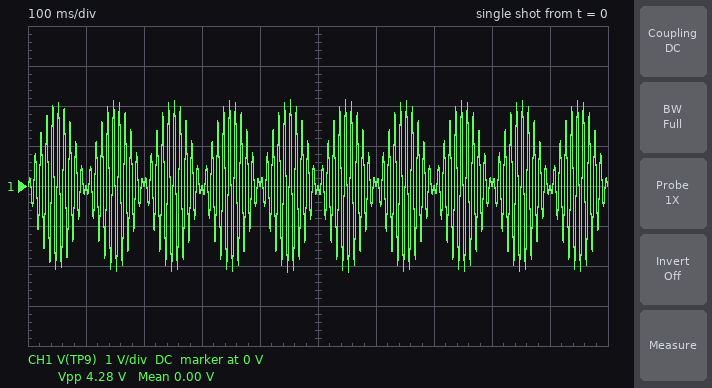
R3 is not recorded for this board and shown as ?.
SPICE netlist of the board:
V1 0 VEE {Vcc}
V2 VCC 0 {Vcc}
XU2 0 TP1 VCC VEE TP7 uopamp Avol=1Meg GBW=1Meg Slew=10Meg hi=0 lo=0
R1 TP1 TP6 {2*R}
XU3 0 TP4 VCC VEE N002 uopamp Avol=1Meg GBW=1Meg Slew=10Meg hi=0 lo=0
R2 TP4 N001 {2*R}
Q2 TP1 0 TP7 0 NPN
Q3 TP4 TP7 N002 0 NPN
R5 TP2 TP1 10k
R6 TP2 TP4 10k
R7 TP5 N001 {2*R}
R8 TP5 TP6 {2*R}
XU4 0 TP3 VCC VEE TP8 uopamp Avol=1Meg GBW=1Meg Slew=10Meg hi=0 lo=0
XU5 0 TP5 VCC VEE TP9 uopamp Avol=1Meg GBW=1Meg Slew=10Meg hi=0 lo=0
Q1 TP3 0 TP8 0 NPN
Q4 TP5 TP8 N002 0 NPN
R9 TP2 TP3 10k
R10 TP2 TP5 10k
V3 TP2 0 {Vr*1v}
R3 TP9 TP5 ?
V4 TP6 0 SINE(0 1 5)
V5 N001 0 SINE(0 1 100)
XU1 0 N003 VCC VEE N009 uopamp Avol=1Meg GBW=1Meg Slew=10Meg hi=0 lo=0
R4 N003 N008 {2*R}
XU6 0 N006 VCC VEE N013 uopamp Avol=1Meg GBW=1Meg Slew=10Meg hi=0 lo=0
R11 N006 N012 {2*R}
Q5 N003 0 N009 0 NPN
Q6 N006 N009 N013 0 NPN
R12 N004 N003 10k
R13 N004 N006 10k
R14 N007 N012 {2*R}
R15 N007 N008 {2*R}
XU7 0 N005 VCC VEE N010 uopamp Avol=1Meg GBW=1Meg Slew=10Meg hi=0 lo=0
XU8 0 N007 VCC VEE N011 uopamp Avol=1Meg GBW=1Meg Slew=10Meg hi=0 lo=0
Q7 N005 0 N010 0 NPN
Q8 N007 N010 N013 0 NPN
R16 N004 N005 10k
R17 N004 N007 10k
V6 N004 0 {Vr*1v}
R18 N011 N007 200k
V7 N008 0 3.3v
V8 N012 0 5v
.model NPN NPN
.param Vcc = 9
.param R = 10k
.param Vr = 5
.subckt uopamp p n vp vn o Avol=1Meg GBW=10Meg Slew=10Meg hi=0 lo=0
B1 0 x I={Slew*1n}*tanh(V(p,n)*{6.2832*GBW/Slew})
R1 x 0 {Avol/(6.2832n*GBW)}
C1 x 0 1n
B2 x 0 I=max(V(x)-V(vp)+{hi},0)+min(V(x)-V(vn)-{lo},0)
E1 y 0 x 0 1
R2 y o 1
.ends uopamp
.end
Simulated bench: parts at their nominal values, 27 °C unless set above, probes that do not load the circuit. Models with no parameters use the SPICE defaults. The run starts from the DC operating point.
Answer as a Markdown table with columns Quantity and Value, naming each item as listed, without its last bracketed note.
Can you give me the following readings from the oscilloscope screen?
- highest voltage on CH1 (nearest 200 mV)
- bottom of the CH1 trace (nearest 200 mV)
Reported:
| Quantity | Value |
|---|---|
| highest voltage on CH1 | 2.2 V |
| bottom of the CH1 trace | -2.2 V |
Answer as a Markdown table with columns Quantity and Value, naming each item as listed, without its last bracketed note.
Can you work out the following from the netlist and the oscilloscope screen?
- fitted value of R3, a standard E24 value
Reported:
| Quantity | Value |
|---|---|
| fitted value of R3, a standard E24 value | 430 kΩ |
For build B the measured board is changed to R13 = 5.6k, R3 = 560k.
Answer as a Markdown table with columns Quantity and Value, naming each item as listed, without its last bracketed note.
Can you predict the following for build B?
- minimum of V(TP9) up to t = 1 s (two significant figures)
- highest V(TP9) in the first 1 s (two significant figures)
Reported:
| Quantity | Value |
|---|---|
| minimum of V(TP9) up to t = 1 s | -2.8 V |
| highest V(TP9) in the first 1 s | 2.8 V |
